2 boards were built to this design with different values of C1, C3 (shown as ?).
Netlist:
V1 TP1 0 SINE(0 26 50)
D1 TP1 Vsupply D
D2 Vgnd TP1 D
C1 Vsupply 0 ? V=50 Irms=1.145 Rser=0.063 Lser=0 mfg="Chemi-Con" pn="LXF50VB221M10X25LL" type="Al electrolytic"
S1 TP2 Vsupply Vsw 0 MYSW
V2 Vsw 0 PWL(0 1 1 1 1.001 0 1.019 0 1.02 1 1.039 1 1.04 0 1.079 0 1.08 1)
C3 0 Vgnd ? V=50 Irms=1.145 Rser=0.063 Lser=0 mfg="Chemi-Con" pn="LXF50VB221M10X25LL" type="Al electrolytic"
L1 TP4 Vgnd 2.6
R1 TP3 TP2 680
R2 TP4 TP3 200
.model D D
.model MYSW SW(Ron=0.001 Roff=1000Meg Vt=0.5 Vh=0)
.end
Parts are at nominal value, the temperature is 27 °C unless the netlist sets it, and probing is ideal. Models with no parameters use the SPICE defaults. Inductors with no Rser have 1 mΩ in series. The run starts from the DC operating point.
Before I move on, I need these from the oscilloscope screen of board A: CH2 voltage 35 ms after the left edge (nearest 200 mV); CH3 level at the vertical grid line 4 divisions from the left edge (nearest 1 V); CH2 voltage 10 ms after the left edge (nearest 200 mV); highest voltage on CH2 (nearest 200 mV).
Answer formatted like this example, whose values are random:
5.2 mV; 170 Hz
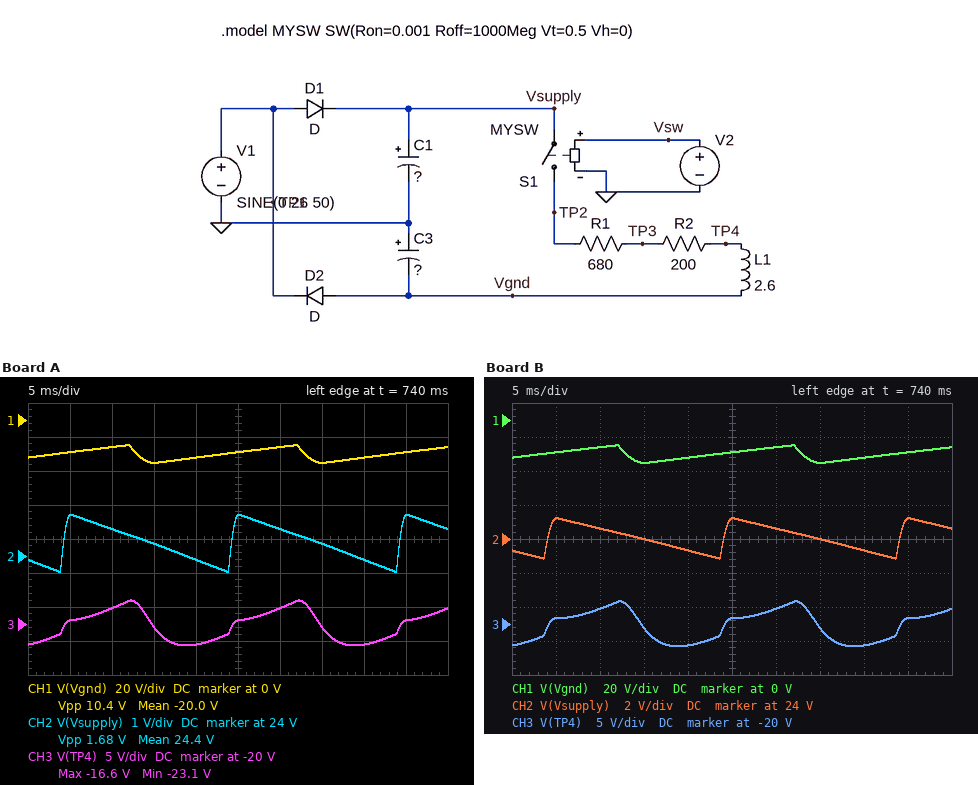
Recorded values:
24.4 V; -23 V; 24.8 V; 25.2 V
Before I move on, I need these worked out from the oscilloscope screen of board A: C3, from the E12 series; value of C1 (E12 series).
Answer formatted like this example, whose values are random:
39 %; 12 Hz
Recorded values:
82 µF; 560 µF
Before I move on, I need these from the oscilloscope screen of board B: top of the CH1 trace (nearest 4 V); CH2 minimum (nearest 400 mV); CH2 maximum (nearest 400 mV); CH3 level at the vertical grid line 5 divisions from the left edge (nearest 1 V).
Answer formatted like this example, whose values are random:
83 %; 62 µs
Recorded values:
-16 V; 22.8 V; 25.2 V; -19 V
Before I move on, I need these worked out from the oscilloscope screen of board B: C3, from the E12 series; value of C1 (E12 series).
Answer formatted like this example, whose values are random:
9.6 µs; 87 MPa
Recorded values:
82 µF; 390 µF
